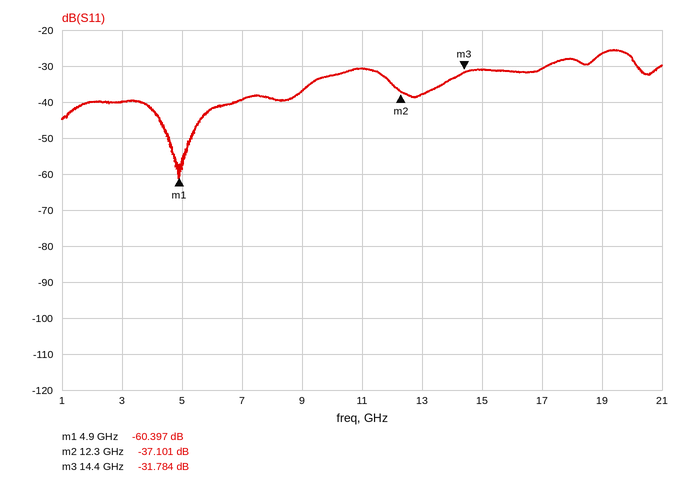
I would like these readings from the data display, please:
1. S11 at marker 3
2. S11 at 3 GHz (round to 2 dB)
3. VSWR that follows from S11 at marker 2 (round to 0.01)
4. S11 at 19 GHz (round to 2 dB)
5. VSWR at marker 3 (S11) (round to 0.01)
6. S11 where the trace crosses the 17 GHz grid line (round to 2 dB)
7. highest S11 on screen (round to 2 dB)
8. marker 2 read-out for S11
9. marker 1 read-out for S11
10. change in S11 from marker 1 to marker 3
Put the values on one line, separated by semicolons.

-31.784 dB; -40 dB; 1.03; -26 dB; 1.05; -30 dB; -26 dB; -37.101 dB; -60.397 dB; 28.613 dB
